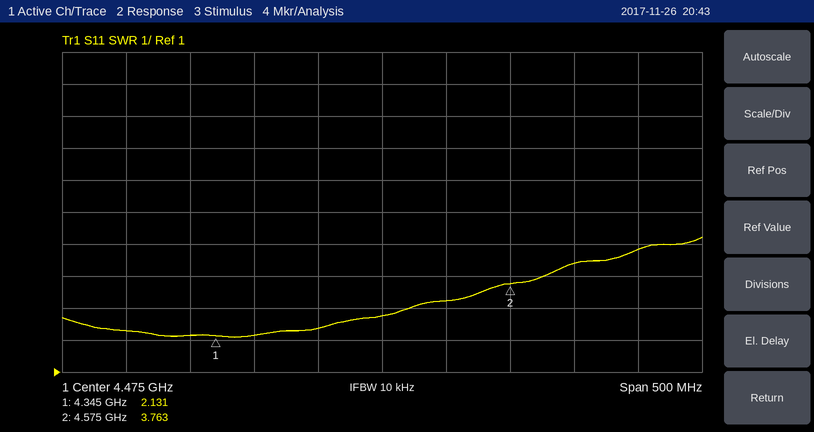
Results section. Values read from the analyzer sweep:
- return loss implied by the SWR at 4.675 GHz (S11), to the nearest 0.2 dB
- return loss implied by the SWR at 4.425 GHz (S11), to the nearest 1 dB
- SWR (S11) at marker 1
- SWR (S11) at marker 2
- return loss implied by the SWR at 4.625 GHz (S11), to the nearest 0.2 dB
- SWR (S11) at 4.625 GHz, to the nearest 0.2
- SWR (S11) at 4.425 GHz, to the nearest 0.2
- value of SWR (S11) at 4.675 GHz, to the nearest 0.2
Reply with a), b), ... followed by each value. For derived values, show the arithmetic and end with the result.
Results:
a) −20 log10((4.8 − 1)/(4.8 + 1)) ≈ 3.67 dB, so 3.6 dB to the nearest 0.2 dB
b) −20 log10((2.4 − 1)/(2.4 + 1)) ≈ 8 dB
c) 2.131
d) 3.763
e) −20 log10((4.4 − 1)/(4.4 + 1)) ≈ 4.0 dB
f) 4.4
g) 2.4
h) 4.8
